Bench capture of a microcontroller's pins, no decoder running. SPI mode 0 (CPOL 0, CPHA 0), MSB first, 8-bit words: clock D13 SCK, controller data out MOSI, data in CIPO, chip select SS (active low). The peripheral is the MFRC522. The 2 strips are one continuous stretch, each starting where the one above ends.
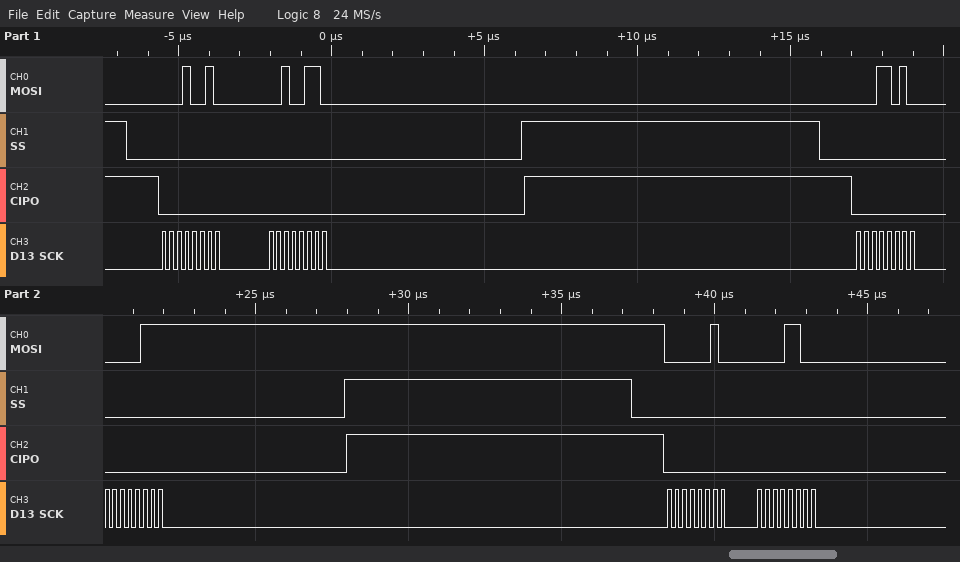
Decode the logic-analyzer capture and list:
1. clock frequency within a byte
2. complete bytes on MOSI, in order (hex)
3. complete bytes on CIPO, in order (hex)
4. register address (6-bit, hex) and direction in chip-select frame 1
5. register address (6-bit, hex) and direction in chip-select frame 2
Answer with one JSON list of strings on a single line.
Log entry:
["4 MHz", "12 26 1A 07 02 0C", "00 00 00 00 00 00", "0x09 write", "0x0D write"]
